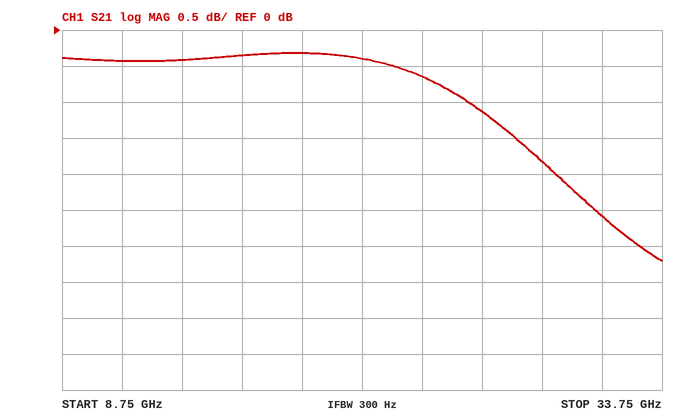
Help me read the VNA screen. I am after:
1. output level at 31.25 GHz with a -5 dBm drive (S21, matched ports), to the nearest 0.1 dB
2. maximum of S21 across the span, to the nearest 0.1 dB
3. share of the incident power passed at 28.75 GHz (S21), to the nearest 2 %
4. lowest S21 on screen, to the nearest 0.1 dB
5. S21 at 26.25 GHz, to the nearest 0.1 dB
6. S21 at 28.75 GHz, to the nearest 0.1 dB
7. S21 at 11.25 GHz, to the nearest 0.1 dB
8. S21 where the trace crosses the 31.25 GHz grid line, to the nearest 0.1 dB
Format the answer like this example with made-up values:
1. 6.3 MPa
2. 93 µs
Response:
1. -7.6 dBm
2. -0.3 dB
3. 66 %
4. -3.2 dB
5. -1.1 dB
6. -1.8 dB
7. -0.4 dB
8. -2.6 dB
